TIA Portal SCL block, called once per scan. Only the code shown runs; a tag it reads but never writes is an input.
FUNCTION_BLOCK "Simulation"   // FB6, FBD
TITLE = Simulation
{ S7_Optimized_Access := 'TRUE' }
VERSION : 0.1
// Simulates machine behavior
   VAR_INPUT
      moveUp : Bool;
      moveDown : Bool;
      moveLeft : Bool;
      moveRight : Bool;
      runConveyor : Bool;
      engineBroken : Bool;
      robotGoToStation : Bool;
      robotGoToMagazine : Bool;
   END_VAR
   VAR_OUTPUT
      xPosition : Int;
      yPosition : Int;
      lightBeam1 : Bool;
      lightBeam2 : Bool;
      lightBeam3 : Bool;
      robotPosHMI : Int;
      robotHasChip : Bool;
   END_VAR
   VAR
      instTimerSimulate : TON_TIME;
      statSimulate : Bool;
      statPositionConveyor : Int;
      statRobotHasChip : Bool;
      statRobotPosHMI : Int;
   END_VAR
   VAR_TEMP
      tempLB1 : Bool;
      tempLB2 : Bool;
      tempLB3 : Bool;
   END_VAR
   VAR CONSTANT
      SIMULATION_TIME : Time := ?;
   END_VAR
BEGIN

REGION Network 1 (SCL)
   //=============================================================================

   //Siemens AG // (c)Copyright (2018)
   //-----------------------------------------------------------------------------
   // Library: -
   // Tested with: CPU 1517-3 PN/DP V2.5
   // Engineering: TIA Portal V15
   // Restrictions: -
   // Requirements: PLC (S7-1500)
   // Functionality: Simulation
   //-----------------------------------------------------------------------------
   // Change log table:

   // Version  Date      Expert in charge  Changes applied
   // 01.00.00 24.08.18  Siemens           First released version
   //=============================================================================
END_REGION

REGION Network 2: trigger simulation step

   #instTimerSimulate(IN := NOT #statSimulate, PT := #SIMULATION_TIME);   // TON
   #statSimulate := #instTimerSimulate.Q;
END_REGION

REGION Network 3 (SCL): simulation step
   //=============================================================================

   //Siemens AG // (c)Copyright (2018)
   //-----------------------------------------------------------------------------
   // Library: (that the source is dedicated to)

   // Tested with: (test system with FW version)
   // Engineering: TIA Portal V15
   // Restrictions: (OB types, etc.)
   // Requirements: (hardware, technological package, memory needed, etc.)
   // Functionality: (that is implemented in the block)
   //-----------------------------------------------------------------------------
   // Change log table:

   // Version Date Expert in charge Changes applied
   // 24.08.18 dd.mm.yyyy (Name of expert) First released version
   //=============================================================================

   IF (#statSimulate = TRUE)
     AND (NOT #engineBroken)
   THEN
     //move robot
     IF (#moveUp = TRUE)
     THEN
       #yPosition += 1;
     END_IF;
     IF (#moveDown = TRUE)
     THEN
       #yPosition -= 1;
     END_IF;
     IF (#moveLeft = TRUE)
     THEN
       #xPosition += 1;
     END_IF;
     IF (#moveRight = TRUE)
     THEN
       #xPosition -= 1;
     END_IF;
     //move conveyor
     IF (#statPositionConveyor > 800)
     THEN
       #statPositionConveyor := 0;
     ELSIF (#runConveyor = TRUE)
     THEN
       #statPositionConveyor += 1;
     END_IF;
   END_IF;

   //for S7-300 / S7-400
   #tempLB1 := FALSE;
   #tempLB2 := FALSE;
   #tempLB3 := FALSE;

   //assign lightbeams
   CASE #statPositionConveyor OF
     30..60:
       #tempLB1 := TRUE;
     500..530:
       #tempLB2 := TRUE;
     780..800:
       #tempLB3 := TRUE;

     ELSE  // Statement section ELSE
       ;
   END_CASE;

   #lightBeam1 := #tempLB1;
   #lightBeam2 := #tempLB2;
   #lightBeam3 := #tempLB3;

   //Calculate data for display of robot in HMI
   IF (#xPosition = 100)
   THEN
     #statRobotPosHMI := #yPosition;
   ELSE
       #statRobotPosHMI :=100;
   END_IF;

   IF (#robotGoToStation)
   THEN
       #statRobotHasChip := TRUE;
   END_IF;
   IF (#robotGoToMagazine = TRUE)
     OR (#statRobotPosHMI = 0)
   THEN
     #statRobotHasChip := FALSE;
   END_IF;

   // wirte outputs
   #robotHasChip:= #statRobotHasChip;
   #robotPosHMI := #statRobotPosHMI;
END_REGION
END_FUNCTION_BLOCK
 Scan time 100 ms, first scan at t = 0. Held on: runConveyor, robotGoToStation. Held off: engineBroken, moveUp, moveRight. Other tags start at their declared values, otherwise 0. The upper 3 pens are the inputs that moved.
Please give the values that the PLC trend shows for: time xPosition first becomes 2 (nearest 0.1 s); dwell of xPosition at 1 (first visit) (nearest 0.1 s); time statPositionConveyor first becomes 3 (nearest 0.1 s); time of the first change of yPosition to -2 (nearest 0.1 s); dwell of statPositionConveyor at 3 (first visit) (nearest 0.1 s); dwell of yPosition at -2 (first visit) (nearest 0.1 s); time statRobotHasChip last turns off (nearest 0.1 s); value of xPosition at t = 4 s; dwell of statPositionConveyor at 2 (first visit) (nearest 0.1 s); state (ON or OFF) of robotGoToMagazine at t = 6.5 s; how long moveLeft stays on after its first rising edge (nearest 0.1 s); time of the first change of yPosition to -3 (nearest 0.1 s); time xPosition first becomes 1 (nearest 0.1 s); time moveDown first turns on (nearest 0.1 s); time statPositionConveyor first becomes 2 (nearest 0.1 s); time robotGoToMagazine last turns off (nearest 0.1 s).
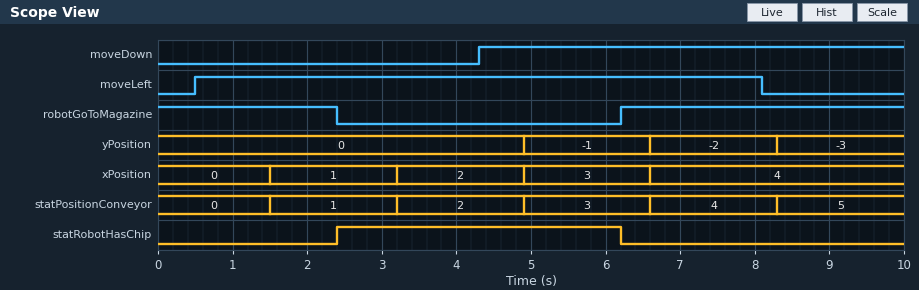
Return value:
3.2 s
1.7 s
4.9 s
6.6 s
1.7 s
1.7 s
6.2 s
2
1.7 s
ON
7.6 s
8.3 s
1.5 s
4.3 s
3.2 s
2.4 s
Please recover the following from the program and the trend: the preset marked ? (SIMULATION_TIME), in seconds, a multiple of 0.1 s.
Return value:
1.5 s
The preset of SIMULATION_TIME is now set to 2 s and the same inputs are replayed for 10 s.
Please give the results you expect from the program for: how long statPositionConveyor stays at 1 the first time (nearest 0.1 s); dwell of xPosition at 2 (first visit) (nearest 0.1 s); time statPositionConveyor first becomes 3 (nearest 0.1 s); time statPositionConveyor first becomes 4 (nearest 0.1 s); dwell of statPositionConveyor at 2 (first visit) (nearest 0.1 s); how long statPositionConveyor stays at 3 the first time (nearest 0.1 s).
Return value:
2.2 s
2.2 s
6.4 s
8.6 s
2.2 s
2.2 s
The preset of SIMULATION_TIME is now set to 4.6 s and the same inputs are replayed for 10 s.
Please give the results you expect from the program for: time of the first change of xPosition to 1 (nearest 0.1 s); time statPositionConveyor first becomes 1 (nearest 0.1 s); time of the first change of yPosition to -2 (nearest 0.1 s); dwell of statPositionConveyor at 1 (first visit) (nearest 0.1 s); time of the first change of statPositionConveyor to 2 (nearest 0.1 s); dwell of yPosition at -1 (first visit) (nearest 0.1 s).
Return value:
4.6 s
4.6 s
9.4 s
4.8 s
9.4 s
4.8 s
